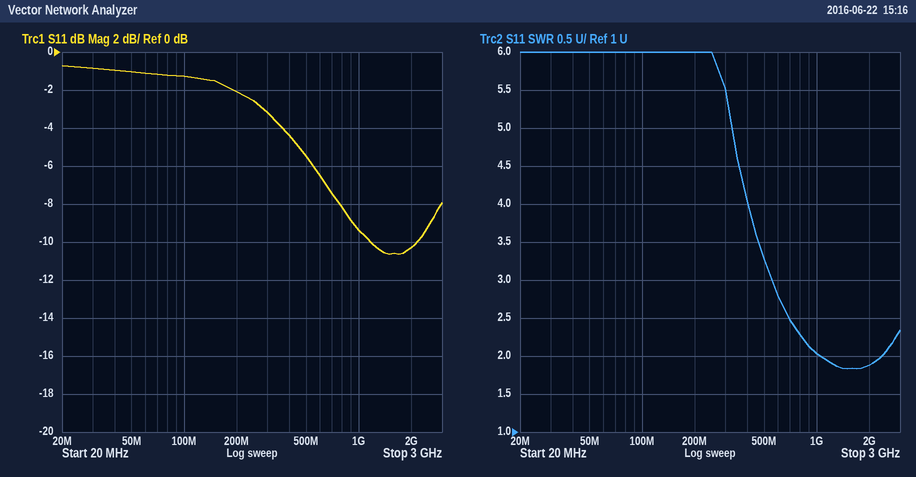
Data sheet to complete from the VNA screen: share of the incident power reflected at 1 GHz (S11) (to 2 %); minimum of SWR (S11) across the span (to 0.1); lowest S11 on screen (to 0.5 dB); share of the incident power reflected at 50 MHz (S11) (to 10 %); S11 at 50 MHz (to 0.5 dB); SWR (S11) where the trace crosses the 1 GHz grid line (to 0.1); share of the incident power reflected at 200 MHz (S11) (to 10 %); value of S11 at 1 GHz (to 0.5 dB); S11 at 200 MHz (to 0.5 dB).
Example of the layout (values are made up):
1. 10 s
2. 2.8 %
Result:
1. 12 %
2. 1.8
3. -10.5 dB
4. 80 %
5. -1.0 dB
6. 2.0
7. 60 %
8. -9.5 dB
9. -2.0 dB
